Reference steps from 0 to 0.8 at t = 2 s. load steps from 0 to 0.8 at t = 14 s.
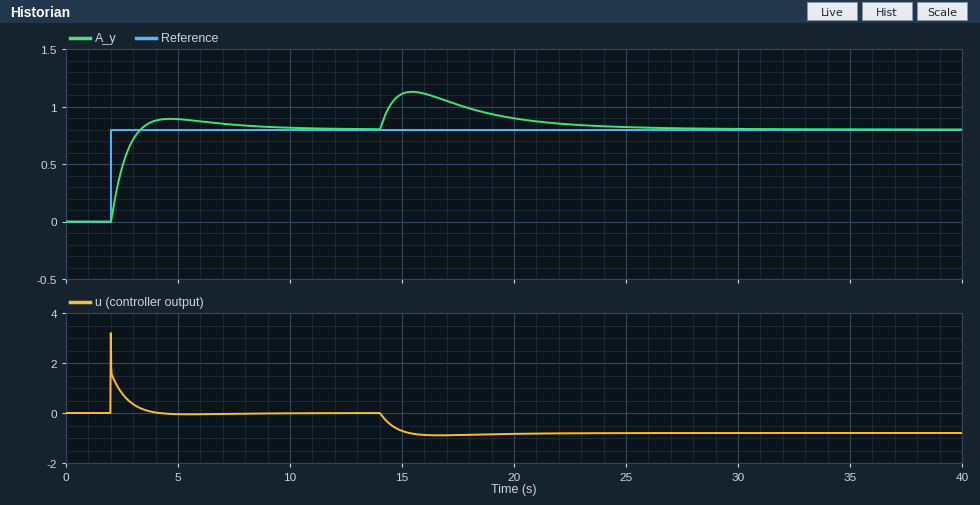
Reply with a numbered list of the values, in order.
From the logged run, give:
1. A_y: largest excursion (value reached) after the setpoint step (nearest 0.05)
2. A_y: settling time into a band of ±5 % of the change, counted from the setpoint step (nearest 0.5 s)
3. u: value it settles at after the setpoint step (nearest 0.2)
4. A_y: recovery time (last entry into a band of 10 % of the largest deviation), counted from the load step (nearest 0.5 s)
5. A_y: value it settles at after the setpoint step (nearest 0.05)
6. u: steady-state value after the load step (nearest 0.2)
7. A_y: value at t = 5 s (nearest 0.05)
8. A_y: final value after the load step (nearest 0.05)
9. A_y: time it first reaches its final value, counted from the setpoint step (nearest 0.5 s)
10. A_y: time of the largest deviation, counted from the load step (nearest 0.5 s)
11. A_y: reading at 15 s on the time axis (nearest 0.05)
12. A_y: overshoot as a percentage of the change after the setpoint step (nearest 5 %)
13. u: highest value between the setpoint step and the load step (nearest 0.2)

1. 0.90
2. 5.5 s
3. 0.0
4. 9.5 s
5. 0.80
6. -0.8
7. 0.90
8. 0.80
9. 1.5 s
10. 1.5 s
11. 1.10
12. 10 %
13. 3.2
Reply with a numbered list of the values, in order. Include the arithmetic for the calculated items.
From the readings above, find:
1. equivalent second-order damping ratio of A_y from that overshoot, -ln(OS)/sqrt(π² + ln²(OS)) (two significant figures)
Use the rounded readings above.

1. ln(0.1) = -2.303; 2.303 / sqrt(9.870 + 5.302) = 0.59
